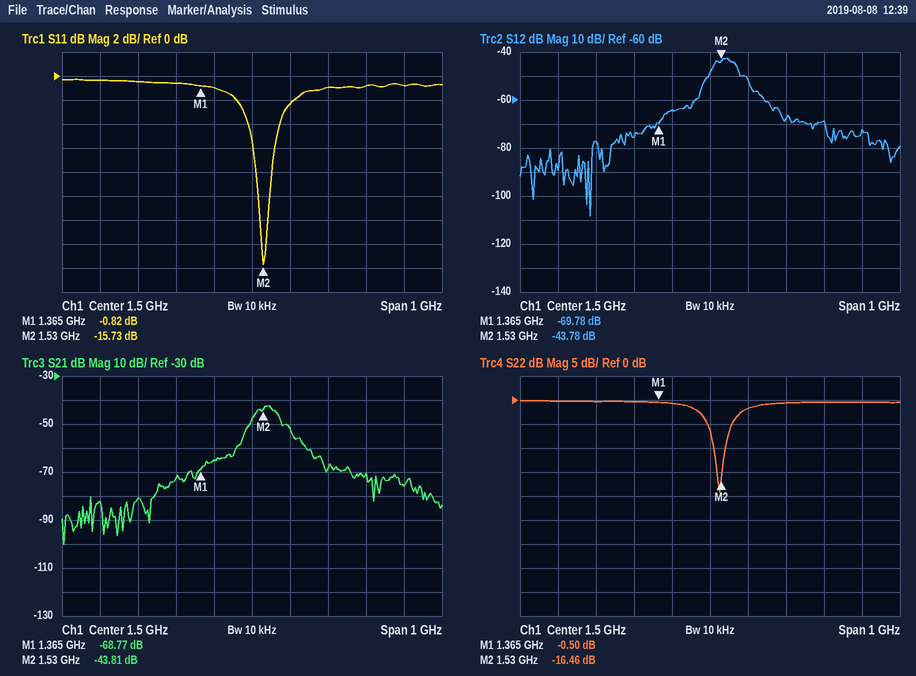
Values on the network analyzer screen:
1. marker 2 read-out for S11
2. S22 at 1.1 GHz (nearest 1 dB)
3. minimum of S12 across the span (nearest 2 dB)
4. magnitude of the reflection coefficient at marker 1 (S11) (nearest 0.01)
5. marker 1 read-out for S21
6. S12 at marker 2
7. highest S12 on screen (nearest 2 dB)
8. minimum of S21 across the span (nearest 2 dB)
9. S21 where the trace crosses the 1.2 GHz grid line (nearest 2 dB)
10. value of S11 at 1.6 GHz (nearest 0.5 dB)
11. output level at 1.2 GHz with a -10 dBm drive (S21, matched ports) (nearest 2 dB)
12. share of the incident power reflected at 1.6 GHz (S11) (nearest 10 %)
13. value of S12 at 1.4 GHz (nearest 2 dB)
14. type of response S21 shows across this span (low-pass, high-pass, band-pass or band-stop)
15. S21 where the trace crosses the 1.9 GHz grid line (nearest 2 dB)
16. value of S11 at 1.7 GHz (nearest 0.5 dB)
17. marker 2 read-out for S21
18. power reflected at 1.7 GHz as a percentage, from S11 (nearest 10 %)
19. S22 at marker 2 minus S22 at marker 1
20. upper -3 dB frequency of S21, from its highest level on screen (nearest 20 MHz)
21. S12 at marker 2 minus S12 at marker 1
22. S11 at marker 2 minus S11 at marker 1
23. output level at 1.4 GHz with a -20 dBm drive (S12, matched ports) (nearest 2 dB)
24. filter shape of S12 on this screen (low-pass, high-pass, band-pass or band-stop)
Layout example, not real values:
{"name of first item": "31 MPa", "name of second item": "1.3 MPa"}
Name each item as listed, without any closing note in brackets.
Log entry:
{"marker 2 read-out for S11": "-15.73 dB", "S22 at 1.1 GHz": "0 dB", "minimum of S12 across the span": "-108 dB", "magnitude of the reflection coefficient at marker 1 (S11)": "0.91", "marker 1 read-out for S21": "-68.77 dB", "S12 at marker 2": "-43.78 dB", "highest S12 on screen": "-42 dB", "minimum of S21 across the span": "-100 dB", "S21 where the trace crosses the 1.2 GHz grid line": "-80 dB", "value of S11 at 1.6 GHz": "-2.5 dB", "output level at 1.2 GHz with a -10 dBm drive (S21, matched ports)": "-90 dBm", "share of the incident power reflected at 1.6 GHz (S11)": "60 %", "value of S12 at 1.4 GHz": "-64 dB", "type of response S21 shows across this span": "band-pass", "S21 where the trace crosses the 1.9 GHz grid line": "-76 dB", "value of S11 at 1.7 GHz": "-1.0 dB", "marker 2 read-out for S21": "-43.81 dB", "power reflected at 1.7 GHz as a percentage, from S11": "80 %", "S22 at marker 2 minus S22 at marker 1": "-15.96 dB", "upper -3 dB frequency of S21, from its highest level on screen": "1.56 GHz", "S12 at marker 2 minus S12 at marker 1": "26.00 dB", "S11 at marker 2 minus S11 at marker 1": "-14.91 dB", "output level at 1.4 GHz with a -20 dBm drive (S12, matched ports)": "-84 dBm", "filter shape of S12 on this screen": "band-pass"}
